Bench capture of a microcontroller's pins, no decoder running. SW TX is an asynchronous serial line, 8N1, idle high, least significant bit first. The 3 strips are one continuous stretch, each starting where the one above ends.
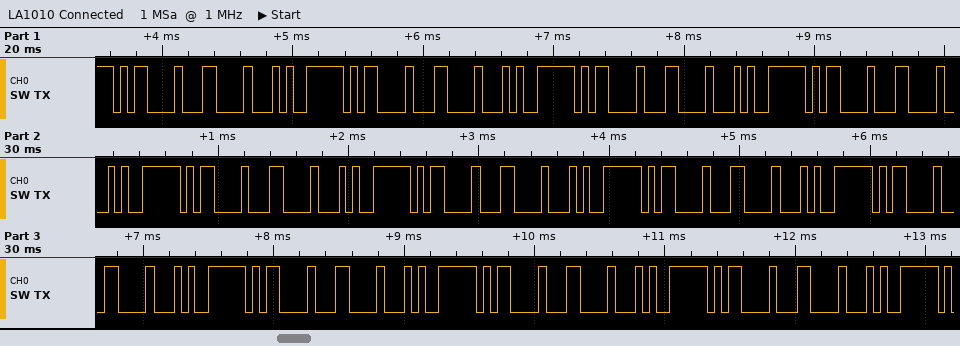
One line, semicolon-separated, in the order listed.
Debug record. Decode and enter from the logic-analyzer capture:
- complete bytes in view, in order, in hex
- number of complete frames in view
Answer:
0x0D 0x0C 0x94 0x0D 0x0C 0x94 0x0D 0x0C 0x94 0x0D 0x0C 0x94 0x0D 0x0C 0x94 0x0D 0x0C 0x94 0x0D 0x0C 0x94 0x0D 0x0C 0x94 0x0D 0x0C 0x94 0x0D 0x0C 0x94 0x0D 0x0C 0x94; 33
